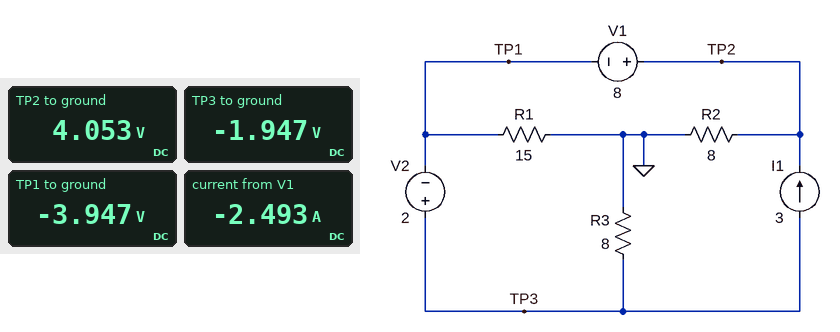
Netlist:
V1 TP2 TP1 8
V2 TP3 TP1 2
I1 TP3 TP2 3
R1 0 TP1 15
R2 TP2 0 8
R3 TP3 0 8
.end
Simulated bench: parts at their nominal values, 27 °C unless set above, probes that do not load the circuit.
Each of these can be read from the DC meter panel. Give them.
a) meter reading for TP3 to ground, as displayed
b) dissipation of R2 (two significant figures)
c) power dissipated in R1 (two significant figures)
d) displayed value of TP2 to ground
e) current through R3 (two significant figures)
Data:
-1.947 V
2.1 W
1.0 W
4.053 V
240 mA
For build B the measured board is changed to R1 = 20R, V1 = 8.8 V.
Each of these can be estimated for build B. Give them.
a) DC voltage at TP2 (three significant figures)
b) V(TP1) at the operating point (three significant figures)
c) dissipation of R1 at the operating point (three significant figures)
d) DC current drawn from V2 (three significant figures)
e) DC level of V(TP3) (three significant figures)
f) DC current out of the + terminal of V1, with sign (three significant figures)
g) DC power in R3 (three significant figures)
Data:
4.30 V
-4.50 V
1.01 W
2.69 A
-2.50 V
-2.46 A
781 mW
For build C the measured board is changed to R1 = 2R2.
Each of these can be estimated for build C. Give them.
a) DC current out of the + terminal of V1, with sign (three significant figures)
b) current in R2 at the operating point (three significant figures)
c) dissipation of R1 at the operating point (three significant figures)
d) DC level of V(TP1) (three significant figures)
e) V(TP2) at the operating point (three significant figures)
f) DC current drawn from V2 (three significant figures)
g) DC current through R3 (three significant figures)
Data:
-2.22 A
778 mA
1.43 W
-1.77 V
6.23 V
3.03 A
28.2 mA
